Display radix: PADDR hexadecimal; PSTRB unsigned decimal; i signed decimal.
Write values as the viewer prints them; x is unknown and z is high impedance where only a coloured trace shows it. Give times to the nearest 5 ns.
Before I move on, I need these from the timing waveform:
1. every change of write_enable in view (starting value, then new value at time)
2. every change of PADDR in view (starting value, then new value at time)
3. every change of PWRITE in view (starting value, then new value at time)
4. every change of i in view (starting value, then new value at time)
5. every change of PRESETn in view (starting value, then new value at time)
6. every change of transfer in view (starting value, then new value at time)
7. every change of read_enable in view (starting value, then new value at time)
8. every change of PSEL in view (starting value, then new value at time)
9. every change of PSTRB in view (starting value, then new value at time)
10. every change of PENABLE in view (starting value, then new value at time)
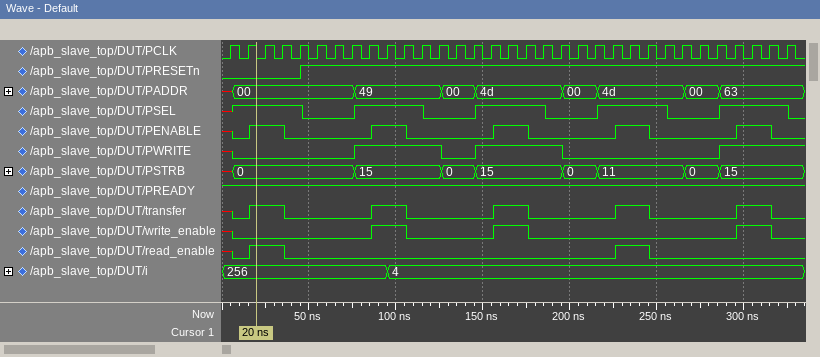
x, 0 at 5 ns, 1 at 85 ns, 0 at 105 ns, 1 at 155 ns, 0 at 175 ns, 1 at 295 ns, 0 at 315 ns
x, 00 at 5 ns, 49 at 75 ns, 00 at 125 ns, 4d at 145 ns, 00 at 195 ns, 4d at 215 ns, 00 at 265 ns, 63 at 285 ns
x, 0 at 5 ns, 1 at 75 ns, 0 at 125 ns, 1 at 145 ns, 0 at 195 ns, 1 at 285 ns
256, 4 at 95 ns
0, 1 at 45 ns
x, 0 at 5 ns, 1 at 15 ns, 0 at 35 ns, 1 at 85 ns, 0 at 105 ns, 1 at 155 ns, 0 at 175 ns, 1 at 225 ns, 0 at 245 ns, 1 at 295 ns, 0 at 315 ns
x, 0 at 5 ns, 1 at 15 ns, 0 at 35 ns, 1 at 225 ns, 0 at 245 ns
x, 1 at 5 ns, 0 at 45 ns, 1 at 75 ns, 0 at 115 ns, 1 at 145 ns, 0 at 185 ns, 1 at 215 ns, 0 at 255 ns, 1 at 285 ns, 0 at 325 ns
x, 0 at 5 ns, 15 at 75 ns, 0 at 125 ns, 15 at 145 ns, 0 at 195 ns, 11 at 215 ns, 0 at 265 ns, 15 at 285 ns
x, 0 at 5 ns, 1 at 15 ns, 0 at 35 ns, 1 at 85 ns, 0 at 105 ns, 1 at 155 ns, 0 at 175 ns, 1 at 225 ns, 0 at 245 ns, 1 at 295 ns, 0 at 315 ns
